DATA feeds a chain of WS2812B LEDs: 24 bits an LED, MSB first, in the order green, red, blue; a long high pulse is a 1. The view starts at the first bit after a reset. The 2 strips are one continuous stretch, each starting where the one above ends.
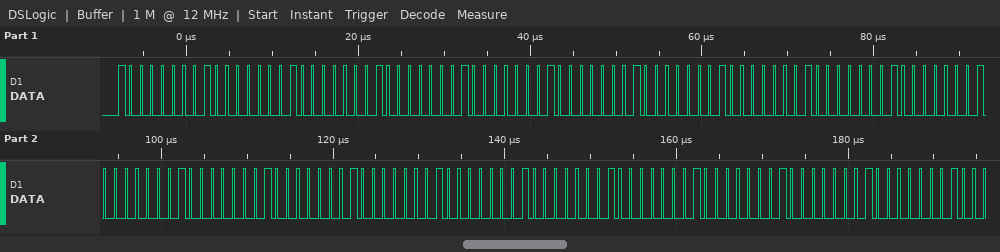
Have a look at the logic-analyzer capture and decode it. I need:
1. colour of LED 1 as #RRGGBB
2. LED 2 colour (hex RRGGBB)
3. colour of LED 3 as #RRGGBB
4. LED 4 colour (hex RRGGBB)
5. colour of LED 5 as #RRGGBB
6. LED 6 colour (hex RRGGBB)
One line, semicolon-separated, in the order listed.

#808080; #808080; #808080; #808080; #808080; #808080
